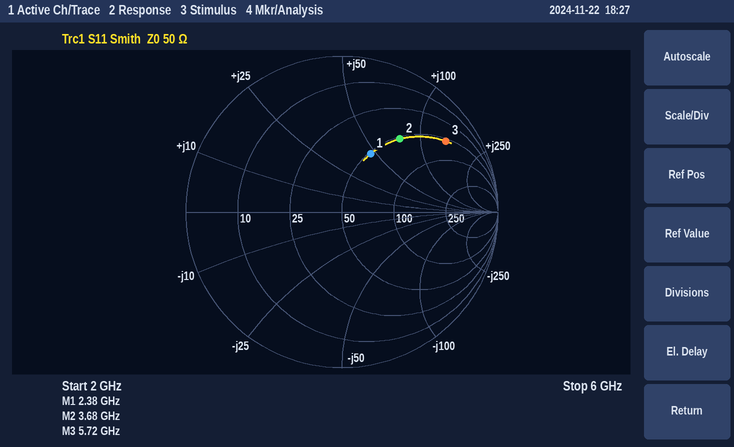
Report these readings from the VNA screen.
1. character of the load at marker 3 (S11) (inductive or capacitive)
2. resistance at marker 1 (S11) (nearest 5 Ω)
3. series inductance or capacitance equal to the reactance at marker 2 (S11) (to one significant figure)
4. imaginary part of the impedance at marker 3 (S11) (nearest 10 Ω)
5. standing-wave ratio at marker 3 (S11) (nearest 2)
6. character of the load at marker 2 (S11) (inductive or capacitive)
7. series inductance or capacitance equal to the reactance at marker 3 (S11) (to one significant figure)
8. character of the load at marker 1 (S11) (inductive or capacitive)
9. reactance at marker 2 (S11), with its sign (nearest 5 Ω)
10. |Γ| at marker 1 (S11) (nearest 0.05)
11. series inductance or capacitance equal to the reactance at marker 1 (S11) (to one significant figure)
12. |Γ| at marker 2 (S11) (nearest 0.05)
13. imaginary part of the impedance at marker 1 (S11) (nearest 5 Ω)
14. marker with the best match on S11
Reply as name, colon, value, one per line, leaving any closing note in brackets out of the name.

character of the load at marker 3 (S11): inductive
resistance at marker 1 (S11): 50 Ω
series inductance or capacitance equal to the reactance at marker 2 (S11): 3 nH
imaginary part of the impedance at marker 3 (S11): +140 Ω
standing-wave ratio at marker 3 (S11): 10
character of the load at marker 2 (S11): inductive
series inductance or capacitance equal to the reactance at marker 3 (S11): 4 nH
character of the load at marker 1 (S11): inductive
reactance at marker 2 (S11), with its sign: +75 Ω
|Γ| at marker 1 (S11): 0.40
series inductance or capacitance equal to the reactance at marker 1 (S11): 3 nH
|Γ| at marker 2 (S11): 0.60
imaginary part of the impedance at marker 1 (S11): +45 Ω
marker with the best match on S11: marker 1
